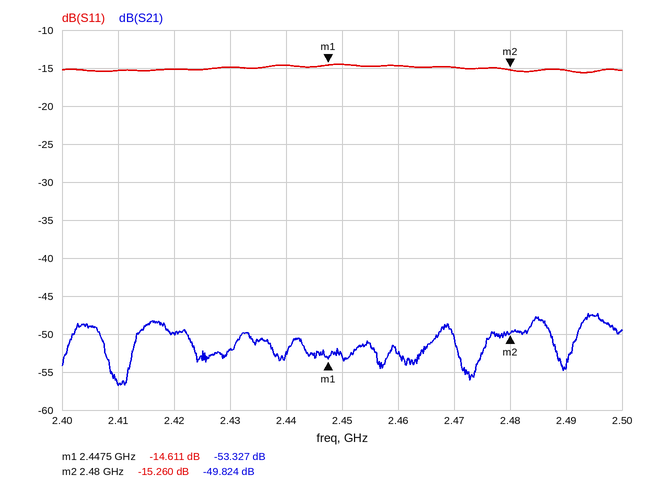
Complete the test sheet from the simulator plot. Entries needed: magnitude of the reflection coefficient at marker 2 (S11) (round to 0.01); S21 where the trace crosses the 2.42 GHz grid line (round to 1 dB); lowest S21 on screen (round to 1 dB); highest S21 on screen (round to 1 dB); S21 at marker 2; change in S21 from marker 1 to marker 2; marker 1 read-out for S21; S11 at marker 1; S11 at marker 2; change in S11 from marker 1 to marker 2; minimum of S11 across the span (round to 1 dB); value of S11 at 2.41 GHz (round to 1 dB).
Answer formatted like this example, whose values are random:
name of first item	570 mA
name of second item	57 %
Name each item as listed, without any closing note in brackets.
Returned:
magnitude of the reflection coefficient at marker 2 (S11)	0.17
S21 where the trace crosses the 2.42 GHz grid line	-50 dB
lowest S21 on screen	-57 dB
highest S21 on screen	-47 dB
S21 at marker 2	-49.824 dB
change in S21 from marker 1 to marker 2	3.503 dB
marker 1 read-out for S21	-53.327 dB
S11 at marker 1	-14.611 dB
S11 at marker 2	-15.260 dB
change in S11 from marker 1 to marker 2	-0.649 dB
minimum of S11 across the span	-16 dB
value of S11 at 2.41 GHz	-15 dB
